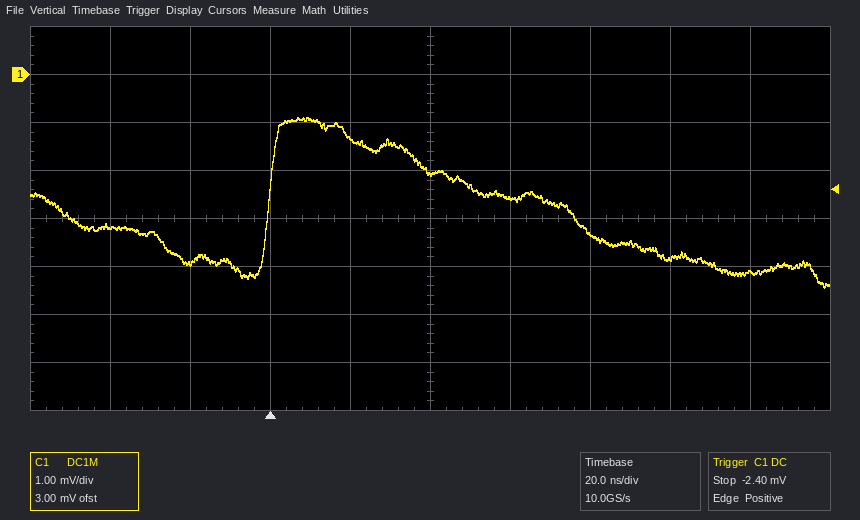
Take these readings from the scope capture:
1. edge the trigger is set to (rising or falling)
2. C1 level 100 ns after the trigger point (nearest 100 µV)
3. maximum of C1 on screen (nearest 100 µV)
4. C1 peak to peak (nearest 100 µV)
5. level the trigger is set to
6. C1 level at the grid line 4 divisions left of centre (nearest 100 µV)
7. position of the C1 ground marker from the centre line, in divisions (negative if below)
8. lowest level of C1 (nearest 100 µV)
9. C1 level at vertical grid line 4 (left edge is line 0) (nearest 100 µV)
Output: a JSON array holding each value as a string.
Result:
["rising", "-3.8 mV", "-900 µV", "3.5 mV", "-2.40 mV", "-3.2 mV", "+3.0 div", "-4.4 mV", "-1.3 mV"]
